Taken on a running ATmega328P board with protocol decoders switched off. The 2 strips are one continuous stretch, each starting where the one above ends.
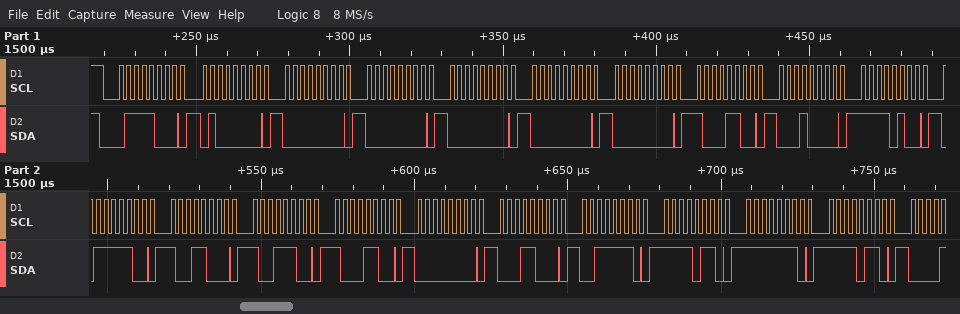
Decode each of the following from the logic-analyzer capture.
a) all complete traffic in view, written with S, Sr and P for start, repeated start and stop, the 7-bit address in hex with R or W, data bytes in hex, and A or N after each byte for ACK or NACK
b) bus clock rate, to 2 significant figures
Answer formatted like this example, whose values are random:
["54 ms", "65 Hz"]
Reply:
["S 3CW A 40 A 00 A 00 A 00 A 00 A 00 A 8C A 10 A F4 A 7C A 98 A 9C A 8C A 00 A 18 A 3E A F6 A FE A F6 A", "400 kHz"]
